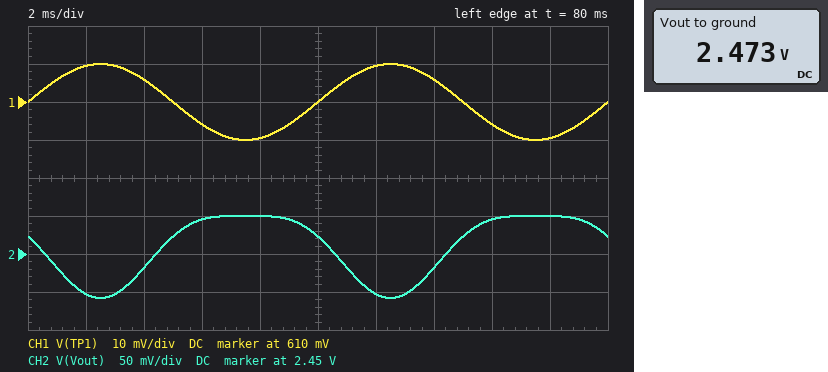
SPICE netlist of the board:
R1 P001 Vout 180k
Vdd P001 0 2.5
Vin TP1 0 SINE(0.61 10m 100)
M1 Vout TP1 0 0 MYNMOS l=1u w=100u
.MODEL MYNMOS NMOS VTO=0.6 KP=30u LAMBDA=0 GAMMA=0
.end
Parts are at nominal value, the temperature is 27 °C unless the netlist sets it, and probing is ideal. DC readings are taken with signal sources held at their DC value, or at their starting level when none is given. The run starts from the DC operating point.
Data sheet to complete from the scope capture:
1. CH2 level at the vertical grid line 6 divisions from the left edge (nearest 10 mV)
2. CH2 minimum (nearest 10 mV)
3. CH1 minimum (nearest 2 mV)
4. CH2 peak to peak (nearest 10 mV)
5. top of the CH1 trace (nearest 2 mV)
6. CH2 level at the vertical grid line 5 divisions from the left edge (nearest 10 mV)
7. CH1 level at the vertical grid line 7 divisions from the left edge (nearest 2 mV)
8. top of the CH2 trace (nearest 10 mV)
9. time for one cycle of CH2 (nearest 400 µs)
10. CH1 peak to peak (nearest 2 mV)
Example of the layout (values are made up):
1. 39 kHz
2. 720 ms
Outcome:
1. 2.40 V
2. 2.39 V
3. 600 mV
4. 110 mV
5. 620 mV
6. 2.47 V
7. 616 mV
8. 2.50 V
9. 10.0 ms
10. 20 mV
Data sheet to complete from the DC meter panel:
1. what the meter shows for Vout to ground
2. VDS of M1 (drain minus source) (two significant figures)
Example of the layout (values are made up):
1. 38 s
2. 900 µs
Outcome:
1. 2.473 V
2. 2.5 V
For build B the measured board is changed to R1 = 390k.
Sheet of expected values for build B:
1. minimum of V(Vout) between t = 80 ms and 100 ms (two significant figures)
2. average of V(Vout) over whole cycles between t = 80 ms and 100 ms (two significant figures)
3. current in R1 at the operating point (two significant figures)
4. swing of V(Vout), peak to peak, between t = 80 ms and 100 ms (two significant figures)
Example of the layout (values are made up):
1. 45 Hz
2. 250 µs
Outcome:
1. 2.3 V
2. 2.4 V
3. 150 nA
4. 230 mV
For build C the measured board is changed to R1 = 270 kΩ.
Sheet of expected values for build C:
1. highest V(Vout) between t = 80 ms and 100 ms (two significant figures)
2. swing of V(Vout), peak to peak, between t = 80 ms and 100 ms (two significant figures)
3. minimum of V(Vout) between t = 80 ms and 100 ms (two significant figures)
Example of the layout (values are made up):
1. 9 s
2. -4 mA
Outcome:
1. 2.5 V
2. 160 mV
3. 2.3 V
